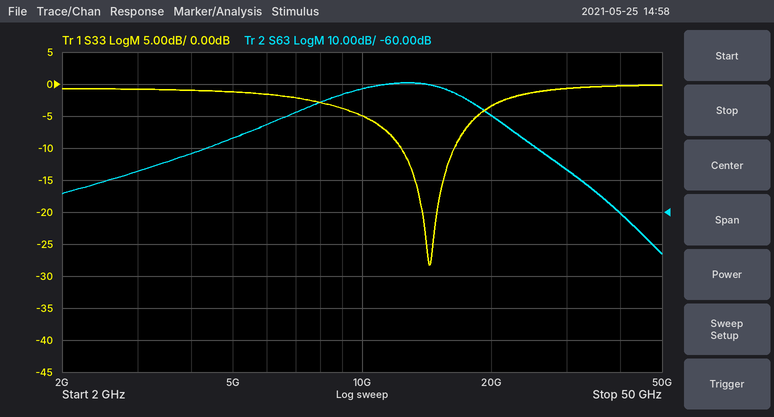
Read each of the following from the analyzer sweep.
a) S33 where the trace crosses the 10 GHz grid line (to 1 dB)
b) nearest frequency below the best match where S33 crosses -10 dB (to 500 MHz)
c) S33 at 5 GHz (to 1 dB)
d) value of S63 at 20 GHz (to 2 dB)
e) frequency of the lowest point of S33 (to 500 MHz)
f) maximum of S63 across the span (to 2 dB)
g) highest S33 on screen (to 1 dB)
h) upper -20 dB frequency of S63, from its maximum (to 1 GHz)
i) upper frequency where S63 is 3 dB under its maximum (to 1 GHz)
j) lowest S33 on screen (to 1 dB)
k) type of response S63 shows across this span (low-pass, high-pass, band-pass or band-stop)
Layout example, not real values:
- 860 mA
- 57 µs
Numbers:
- -5 dB
- 12.5 GHz
- -1 dB
- -30 dB
- 14.5 GHz
- -20 dB
- 0 dB
- 25 GHz
- 16 GHz
- -28 dB
- band-pass
